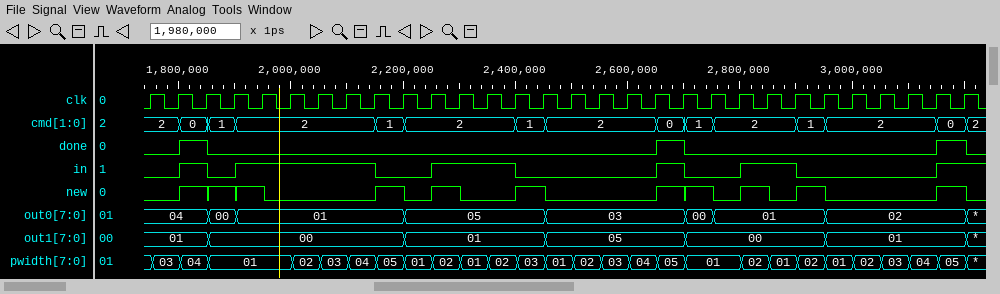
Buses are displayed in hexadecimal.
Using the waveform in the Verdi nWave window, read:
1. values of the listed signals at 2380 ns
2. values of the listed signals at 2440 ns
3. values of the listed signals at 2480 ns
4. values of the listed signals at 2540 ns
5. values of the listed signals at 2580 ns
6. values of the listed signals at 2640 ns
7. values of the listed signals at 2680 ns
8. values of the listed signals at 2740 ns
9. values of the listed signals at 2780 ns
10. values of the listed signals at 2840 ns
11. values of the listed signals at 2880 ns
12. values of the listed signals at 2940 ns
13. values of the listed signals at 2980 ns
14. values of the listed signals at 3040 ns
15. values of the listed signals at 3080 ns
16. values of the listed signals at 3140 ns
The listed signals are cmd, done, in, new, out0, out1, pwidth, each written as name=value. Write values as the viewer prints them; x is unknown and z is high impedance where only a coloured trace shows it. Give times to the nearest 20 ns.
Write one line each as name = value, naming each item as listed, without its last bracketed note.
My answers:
values of the listed signals at 2380 ns = cmd=2, done=0, in=1, new=0, out0=05, out1=01, pwidth=02
values of the listed signals at 2440 ns = cmd=1, done=0, in=0, new=1, out0=05, out1=01, pwidth=03
values of the listed signals at 2480 ns = cmd=2, done=0, in=0, new=0, out0=03, out1=05, pwidth=01
values of the listed signals at 2540 ns = cmd=2, done=0, in=0, new=0, out0=03, out1=05, pwidth=02
values of the listed signals at 2580 ns = cmd=2, done=0, in=0, new=0, out0=03, out1=05, pwidth=03
values of the listed signals at 2640 ns = cmd=2, done=0, in=0, new=0, out0=03, out1=05, pwidth=04
values of the listed signals at 2680 ns = cmd=0, done=1, in=1, new=1, out0=03, out1=05, pwidth=05
values of the listed signals at 2740 ns = cmd=1, done=0, in=0, new=1, out0=00, out1=00, pwidth=01
values of the listed signals at 2780 ns = cmd=2, done=0, in=0, new=0, out0=01, out1=00, pwidth=01
values of the listed signals at 2840 ns = cmd=2, done=0, in=1, new=1, out0=01, out1=00, pwidth=02
values of the listed signals at 2880 ns = cmd=2, done=0, in=1, new=0, out0=01, out1=00, pwidth=01
values of the listed signals at 2940 ns = cmd=1, done=0, in=0, new=1, out0=01, out1=00, pwidth=02
values of the listed signals at 2980 ns = cmd=2, done=0, in=0, new=0, out0=02, out1=01, pwidth=01
values of the listed signals at 3040 ns = cmd=2, done=0, in=0, new=0, out0=02, out1=01, pwidth=02
values of the listed signals at 3080 ns = cmd=2, done=0, in=0, new=0, out0=02, out1=01, pwidth=03
values of the listed signals at 3140 ns = cmd=2, done=0, in=0, new=0, out0=02, out1=01, pwidth=04
